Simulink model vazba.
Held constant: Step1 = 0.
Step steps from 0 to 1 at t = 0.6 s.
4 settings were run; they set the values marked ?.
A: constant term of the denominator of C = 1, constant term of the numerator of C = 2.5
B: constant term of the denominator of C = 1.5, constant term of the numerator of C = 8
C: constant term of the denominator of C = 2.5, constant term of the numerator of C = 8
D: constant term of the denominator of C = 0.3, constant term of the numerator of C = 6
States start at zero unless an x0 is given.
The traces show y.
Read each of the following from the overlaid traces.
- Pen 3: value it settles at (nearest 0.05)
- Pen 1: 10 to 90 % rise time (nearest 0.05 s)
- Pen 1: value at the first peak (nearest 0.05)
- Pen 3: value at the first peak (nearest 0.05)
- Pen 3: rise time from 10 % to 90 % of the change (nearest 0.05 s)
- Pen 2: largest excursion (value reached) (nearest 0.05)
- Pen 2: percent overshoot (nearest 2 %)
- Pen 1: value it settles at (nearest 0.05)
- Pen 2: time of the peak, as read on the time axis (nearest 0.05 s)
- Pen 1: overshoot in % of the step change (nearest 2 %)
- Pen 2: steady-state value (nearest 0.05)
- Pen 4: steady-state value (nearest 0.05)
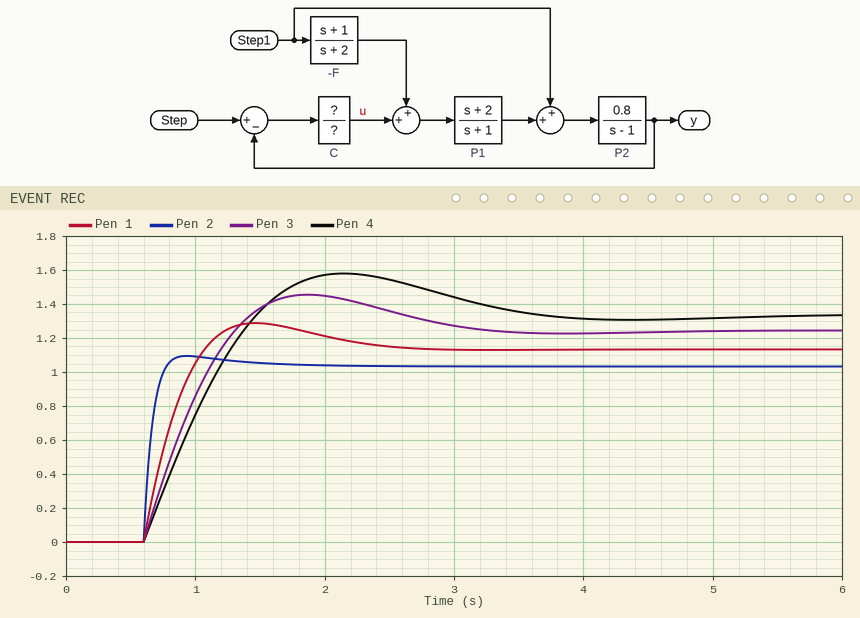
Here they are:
1.25
0.35 s
1.30
1.45
0.55 s
1.10
6 %
1.15
0.95 s
14 %
1.05
1.35
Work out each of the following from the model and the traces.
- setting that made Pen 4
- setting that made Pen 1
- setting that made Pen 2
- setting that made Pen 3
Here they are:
A
B
D
C
